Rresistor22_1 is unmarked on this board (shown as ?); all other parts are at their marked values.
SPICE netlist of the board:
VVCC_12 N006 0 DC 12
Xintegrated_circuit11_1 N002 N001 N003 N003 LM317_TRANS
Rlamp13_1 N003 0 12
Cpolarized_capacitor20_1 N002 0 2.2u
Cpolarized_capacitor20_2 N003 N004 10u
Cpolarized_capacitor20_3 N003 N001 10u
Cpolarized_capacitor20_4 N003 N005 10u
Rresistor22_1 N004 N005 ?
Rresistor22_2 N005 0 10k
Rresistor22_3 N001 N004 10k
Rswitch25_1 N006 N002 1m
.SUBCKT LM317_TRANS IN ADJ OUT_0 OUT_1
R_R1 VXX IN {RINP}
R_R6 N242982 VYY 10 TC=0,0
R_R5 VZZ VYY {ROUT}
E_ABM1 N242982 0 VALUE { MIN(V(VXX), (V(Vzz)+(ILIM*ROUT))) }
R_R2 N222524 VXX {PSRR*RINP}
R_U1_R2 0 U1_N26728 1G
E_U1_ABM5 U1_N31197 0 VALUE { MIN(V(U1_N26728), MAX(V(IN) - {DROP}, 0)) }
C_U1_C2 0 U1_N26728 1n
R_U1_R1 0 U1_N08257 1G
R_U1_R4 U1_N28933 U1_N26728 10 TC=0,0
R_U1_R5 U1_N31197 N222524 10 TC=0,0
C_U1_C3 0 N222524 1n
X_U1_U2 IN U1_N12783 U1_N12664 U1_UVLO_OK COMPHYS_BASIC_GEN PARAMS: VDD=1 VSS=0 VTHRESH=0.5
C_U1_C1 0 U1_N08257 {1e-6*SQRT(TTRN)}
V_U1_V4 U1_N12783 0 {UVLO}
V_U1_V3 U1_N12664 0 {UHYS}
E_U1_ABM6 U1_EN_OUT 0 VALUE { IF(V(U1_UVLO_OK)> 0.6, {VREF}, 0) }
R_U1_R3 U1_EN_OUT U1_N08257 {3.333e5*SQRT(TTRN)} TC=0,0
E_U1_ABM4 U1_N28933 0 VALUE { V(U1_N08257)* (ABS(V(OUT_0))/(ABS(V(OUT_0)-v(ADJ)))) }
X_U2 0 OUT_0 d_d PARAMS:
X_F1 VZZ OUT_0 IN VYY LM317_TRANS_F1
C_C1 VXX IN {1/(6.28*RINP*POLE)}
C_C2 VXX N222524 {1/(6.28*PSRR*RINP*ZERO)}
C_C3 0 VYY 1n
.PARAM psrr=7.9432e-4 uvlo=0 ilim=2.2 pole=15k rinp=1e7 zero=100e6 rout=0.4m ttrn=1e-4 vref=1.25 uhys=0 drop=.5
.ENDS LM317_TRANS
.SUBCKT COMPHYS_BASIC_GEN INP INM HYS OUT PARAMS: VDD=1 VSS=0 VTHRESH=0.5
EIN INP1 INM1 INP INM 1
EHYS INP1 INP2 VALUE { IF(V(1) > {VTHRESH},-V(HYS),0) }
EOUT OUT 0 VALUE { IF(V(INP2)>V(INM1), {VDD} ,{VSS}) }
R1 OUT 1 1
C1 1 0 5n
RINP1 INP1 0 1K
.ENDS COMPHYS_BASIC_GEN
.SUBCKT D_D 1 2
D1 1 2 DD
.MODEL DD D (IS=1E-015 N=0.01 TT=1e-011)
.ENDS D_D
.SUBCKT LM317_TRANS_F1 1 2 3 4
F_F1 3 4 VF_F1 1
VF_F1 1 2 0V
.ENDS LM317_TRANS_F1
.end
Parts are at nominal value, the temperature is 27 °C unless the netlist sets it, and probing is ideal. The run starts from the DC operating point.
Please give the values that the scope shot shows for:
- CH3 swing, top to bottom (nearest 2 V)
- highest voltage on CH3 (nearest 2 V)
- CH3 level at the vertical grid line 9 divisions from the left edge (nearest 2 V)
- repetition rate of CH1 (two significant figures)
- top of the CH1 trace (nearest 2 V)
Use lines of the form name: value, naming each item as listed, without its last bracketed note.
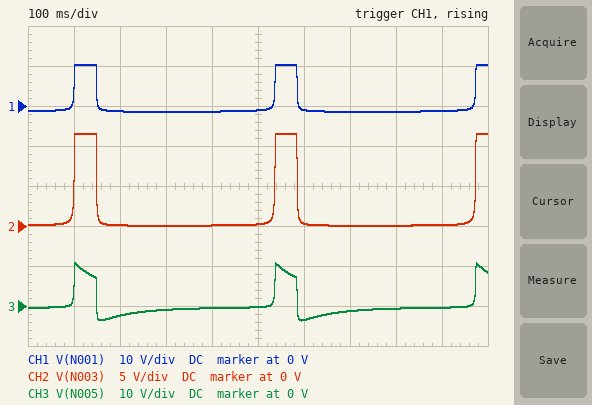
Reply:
CH3 swing, top to bottom: 14 V
highest voltage on CH3: 10 V
CH3 level at the vertical grid line 9 divisions from the left edge: 0 V
repetition rate of CH1: 2.3 Hz
top of the CH1 trace: 10 V
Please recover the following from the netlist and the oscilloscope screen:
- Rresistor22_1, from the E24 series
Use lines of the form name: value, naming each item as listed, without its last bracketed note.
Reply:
Rresistor22_1, from the E24 series: 20 kΩ
